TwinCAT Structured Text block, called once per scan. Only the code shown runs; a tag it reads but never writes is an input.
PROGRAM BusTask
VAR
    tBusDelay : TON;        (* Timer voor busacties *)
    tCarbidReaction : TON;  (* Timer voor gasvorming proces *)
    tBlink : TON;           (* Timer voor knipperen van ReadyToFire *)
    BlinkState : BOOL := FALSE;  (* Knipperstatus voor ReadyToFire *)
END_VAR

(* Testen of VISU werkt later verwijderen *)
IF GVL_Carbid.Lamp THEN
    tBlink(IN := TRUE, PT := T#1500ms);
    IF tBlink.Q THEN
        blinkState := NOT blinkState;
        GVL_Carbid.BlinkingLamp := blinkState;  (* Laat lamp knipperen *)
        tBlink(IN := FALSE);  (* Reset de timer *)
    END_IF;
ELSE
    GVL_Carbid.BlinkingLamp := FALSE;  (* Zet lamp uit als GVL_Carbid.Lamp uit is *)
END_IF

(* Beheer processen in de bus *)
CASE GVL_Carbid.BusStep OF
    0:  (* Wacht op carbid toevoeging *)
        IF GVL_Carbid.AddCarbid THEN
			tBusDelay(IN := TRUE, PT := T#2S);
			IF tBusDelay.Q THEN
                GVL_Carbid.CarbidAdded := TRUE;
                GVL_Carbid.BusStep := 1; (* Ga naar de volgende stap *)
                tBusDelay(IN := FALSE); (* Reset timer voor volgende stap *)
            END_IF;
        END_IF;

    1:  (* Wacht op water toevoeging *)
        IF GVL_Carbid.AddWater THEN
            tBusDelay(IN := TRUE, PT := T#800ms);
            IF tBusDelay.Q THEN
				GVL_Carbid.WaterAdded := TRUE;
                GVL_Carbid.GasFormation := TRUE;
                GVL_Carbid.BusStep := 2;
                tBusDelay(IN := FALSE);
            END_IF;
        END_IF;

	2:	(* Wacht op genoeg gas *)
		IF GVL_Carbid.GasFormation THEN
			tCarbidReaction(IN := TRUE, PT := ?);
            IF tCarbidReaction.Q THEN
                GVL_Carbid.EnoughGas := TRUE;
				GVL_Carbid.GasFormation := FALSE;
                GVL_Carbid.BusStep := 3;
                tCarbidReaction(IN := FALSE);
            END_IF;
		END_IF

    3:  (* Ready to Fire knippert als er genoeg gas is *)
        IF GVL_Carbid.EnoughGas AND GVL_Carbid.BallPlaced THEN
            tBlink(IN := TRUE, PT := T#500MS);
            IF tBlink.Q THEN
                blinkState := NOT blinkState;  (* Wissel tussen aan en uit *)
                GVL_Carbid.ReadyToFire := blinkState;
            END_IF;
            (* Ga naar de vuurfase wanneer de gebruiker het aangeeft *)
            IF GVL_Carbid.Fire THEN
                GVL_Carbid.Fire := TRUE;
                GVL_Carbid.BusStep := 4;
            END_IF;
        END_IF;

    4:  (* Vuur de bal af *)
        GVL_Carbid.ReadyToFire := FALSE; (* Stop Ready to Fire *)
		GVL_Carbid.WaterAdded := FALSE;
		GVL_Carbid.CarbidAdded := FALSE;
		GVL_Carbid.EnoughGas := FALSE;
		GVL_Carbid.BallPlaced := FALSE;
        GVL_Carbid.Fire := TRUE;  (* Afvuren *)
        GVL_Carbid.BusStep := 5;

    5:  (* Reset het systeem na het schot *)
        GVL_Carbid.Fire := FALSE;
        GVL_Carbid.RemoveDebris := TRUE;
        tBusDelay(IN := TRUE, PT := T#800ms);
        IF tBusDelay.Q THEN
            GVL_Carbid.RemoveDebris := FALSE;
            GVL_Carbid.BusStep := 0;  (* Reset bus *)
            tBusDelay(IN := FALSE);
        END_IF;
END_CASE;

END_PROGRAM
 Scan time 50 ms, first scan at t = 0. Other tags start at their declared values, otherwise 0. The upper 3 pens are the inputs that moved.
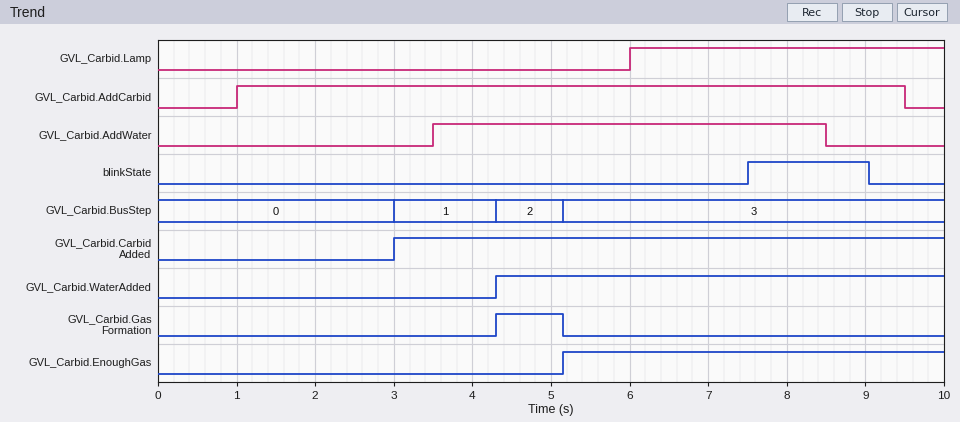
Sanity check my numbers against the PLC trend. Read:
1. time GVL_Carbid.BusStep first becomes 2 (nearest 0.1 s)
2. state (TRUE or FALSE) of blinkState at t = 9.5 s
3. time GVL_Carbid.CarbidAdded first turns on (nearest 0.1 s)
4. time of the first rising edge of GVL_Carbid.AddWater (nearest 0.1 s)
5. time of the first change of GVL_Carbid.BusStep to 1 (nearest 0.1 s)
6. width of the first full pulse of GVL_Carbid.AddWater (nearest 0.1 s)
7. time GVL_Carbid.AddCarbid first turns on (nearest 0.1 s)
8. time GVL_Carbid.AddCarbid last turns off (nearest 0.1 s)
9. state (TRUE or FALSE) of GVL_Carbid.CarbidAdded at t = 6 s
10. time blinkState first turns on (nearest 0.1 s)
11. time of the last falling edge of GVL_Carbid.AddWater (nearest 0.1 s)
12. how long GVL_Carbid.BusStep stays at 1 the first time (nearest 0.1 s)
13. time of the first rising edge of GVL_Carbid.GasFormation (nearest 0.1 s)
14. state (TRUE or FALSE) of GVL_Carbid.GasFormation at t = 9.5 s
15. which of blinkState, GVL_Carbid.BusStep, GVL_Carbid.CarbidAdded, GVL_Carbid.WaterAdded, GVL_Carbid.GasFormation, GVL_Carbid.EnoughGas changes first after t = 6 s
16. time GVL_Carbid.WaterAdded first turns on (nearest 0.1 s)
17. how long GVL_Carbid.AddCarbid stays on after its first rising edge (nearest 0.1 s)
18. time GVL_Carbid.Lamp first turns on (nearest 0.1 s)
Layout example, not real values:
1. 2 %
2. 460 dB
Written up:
1. 4.3 s
2. FALSE
3. 3.0 s
4. 3.5 s
5. 3.0 s
6. 5.0 s
7. 1.0 s
8. 9.5 s
9. TRUE
10. 7.5 s
11. 8.5 s
12. 1.3 s
13. 4.3 s
14. FALSE
15. blinkState
16. 4.3 s
17. 8.5 s
18. 6.0 s
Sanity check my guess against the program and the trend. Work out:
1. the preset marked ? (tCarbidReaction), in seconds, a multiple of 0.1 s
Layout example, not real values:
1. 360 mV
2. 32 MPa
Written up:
1. 0.8 s
